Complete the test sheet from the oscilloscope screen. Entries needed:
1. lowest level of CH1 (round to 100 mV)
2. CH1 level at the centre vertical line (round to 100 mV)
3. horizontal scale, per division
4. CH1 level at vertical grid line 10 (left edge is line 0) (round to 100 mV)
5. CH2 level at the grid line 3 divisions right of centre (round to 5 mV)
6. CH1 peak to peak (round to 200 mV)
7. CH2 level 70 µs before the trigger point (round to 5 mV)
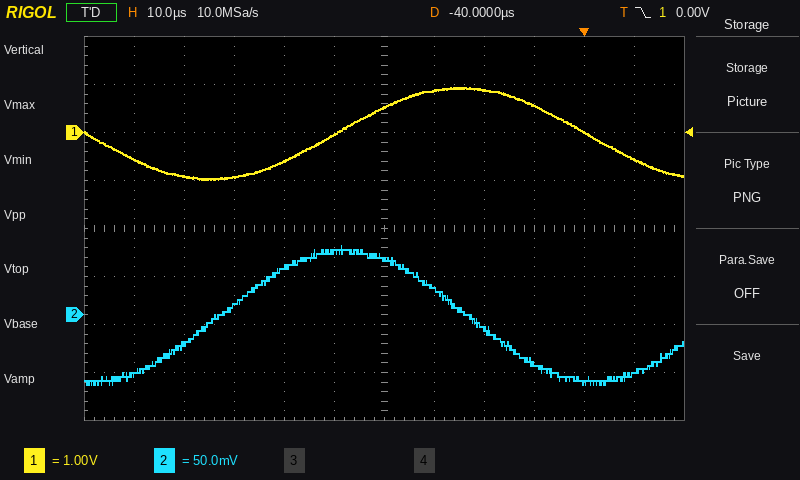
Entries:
-1.0 V
500 mV
10 µs
0.0 V
-50 mV
2.0 V
10 mV
